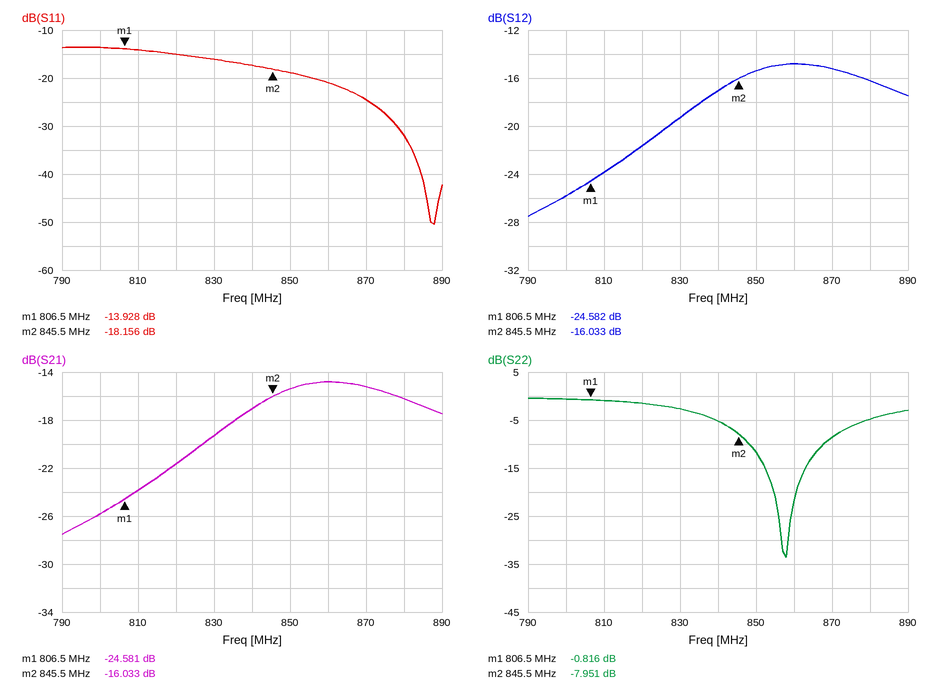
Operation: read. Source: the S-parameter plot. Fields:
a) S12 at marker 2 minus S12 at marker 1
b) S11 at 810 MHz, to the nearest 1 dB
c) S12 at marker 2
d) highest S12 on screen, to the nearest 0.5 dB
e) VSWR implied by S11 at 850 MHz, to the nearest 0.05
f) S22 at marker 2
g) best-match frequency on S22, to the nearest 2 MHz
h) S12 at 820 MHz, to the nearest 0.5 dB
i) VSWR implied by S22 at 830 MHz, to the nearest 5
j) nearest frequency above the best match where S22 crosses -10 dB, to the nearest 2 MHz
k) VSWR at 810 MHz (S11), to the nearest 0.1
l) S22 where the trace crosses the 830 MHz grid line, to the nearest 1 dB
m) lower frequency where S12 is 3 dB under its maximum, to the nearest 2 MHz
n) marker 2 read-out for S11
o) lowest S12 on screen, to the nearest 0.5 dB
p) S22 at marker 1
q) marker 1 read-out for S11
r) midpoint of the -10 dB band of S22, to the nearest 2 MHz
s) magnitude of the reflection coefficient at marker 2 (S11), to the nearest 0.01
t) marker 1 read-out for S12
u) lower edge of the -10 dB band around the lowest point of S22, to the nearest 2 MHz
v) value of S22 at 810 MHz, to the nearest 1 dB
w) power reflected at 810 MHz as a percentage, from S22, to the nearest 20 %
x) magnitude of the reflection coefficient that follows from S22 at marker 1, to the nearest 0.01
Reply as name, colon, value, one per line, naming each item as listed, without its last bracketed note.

S12 at marker 2 minus S12 at marker 1: 8.549 dB
S11 at 810 MHz, to the nearest 1 dB: -14 dB
S12 at marker 2: -16.033 dB
highest S12 on screen, to the nearest 0.5 dB: -15.0 dB
VSWR implied by S11 at 850 MHz, to the nearest 0.05: 1.25
S22 at marker 2: -7.951 dB
best-match frequency on S22, to the nearest 2 MHz: 858 MHz
S12 at 820 MHz, to the nearest 0.5 dB: -21.5 dB
VSWR implied by S22 at 830 MHz, to the nearest 5: 5
nearest frequency above the best match where S22 crosses -10 dB, to the nearest 2 MHz: 868 MHz
VSWR at 810 MHz (S11), to the nearest 0.1: 1.5
S22 where the trace crosses the 830 MHz grid line, to the nearest 1 dB: -3 dB
lower frequency where S12 is 3 dB under its maximum, to the nearest 2 MHz: 836 MHz
marker 2 read-out for S11: -18.156 dB
lowest S12 on screen, to the nearest 0.5 dB: -27.5 dB
S22 at marker 1: -0.816 dB
marker 1 read-out for S11: -13.928 dB
midpoint of the -10 dB band of S22, to the nearest 2 MHz: 858 MHz
magnitude of the reflection coefficient at marker 2 (S11), to the nearest 0.01: 0.12
marker 1 read-out for S12: -24.582 dB
lower edge of the -10 dB band around the lowest point of S22, to the nearest 2 MHz: 848 MHz
value of S22 at 810 MHz, to the nearest 1 dB: -1 dB
power reflected at 810 MHz as a percentage, from S22, to the nearest 20 %: 80 %
magnitude of the reflection coefficient that follows from S22 at marker 1, to the nearest 0.01: 0.91
